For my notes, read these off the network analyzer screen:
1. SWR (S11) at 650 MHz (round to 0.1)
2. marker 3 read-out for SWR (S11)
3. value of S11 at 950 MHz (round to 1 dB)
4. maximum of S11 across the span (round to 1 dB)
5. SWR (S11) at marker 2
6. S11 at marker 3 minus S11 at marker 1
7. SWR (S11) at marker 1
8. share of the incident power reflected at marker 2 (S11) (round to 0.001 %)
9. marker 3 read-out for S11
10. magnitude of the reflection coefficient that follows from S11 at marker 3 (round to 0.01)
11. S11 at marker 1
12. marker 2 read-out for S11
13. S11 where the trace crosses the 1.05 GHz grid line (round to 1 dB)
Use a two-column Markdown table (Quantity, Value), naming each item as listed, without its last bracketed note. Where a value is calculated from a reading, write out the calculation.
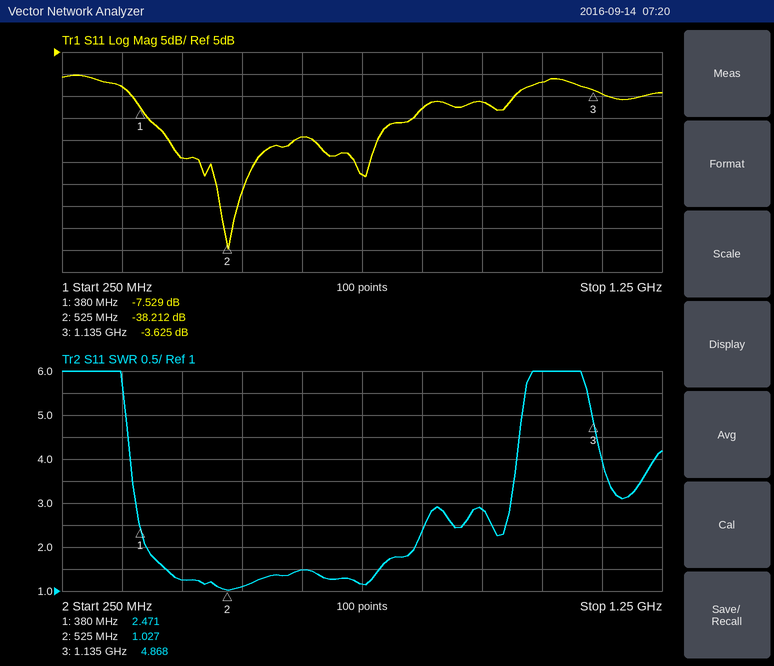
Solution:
| Quantity | Value |
|---|---|
| SWR (S11) at 650 MHz | 1.5 |
| marker 3 read-out for SWR | 4.868 |
| value of S11 at 950 MHz | -6 dB |
| maximum of S11 across the span | 0 dB |
| SWR (S11) at marker 2 | 1.027 |
| S11 at marker 3 minus S11 at marker 1 | -3.625 − (-7.529) = 3.904 dB |
| SWR (S11) at marker 1 | 2.471 |
| share of the incident power reflected at marker 2 (S11) | 10^(-38.212/10) ≈ 0.015 % |
| marker 3 read-out for S11 | -3.625 dB |
| magnitude of the reflection coefficient that follows from S11 at marker 3 | 10^(-3.625/20) ≈ 0.66 |
| S11 at marker 1 | -7.529 dB |
| marker 2 read-out for S11 | -38.212 dB |
| S11 where the trace crosses the 1.05 GHz grid line | -2 dB |
